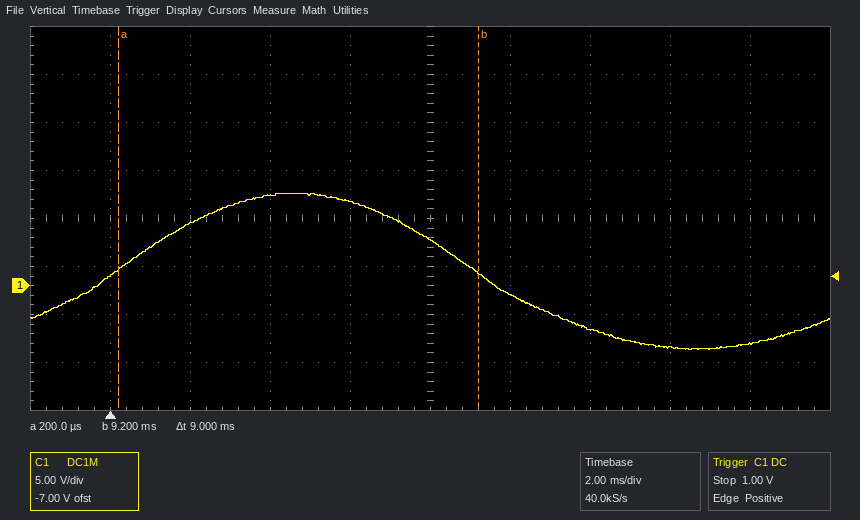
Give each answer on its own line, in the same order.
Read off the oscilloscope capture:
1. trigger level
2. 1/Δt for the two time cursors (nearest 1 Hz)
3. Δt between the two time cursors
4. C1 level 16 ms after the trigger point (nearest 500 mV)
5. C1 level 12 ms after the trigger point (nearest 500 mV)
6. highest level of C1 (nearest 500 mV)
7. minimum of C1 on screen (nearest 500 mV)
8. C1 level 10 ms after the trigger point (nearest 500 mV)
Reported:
1.00 V
111 Hz
9 ms
-6.0 V
-4.5 V
9.5 V
-6.5 V
-1.0 V
